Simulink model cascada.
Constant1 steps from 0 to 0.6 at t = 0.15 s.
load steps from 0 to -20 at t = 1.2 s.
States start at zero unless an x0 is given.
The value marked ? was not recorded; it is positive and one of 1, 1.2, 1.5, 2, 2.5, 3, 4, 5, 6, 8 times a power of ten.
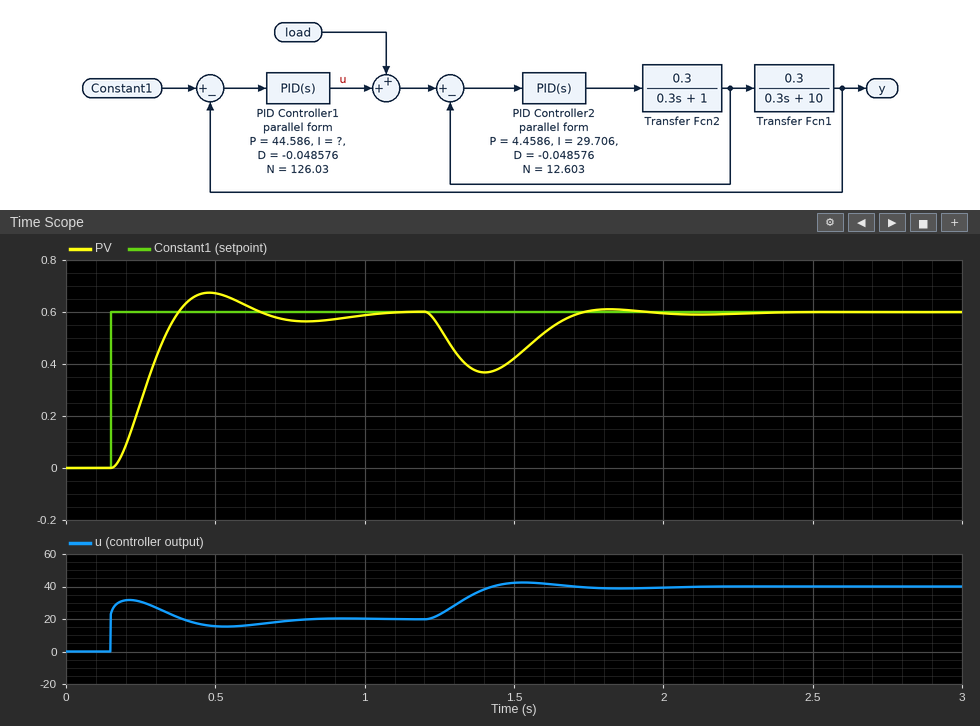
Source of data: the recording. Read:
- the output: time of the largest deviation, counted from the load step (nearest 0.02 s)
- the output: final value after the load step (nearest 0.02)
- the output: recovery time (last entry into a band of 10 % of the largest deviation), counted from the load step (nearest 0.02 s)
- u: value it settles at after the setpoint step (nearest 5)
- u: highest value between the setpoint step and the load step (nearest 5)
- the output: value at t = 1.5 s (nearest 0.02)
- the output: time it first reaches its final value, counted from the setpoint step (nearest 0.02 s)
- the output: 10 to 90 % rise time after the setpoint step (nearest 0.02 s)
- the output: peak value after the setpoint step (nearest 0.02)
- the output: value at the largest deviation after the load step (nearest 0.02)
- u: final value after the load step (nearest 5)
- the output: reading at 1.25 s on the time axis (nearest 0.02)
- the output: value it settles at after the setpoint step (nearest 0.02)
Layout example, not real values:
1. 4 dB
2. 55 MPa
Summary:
1. 0.20 s
2. 0.60
3. 0.48 s
4. 20
5. 30
6. 0.42
7. 0.22 s
8. 0.16 s
9. 0.68
10. 0.36
11. 40
12. 0.54
13. 0.60
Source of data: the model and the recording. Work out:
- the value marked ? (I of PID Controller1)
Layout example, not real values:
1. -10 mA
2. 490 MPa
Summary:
1. 300
